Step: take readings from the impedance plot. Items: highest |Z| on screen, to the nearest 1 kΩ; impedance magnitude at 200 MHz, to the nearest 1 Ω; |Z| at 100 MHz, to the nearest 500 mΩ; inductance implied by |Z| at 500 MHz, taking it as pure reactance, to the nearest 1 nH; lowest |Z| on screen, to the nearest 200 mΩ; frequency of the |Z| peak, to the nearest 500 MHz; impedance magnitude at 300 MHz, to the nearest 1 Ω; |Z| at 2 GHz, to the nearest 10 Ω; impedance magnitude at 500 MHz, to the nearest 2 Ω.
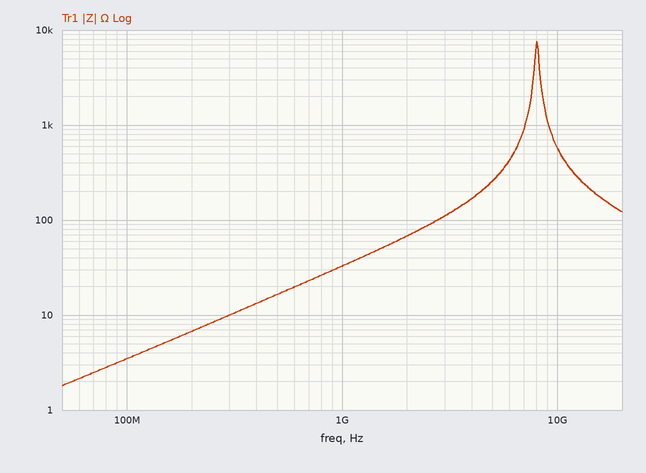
8 kΩ
7 Ω
3.5 Ω
5 nH
1.8 Ω
8.0 GHz
10 Ω
70 Ω
16 Ω
